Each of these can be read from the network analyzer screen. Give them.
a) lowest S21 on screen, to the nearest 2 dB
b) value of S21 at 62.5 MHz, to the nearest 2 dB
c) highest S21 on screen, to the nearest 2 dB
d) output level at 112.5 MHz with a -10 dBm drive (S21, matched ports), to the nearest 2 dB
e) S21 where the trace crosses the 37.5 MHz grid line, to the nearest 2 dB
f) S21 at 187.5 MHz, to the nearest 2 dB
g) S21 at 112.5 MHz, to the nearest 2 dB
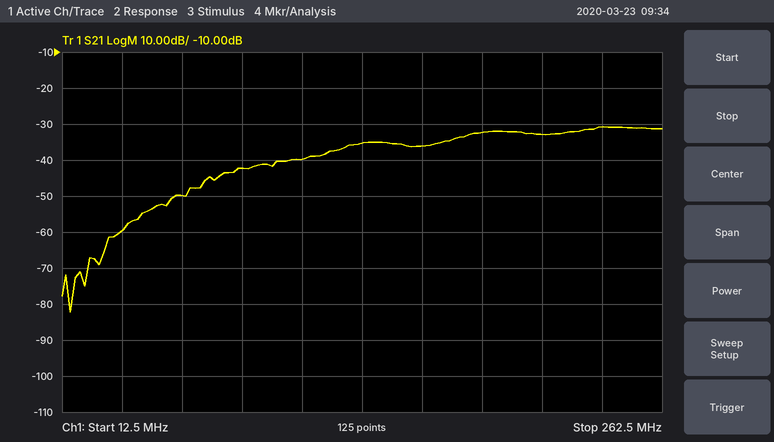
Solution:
-82 dB
-50 dB
-30 dB
-50 dBm
-60 dB
-32 dB
-40 dB
